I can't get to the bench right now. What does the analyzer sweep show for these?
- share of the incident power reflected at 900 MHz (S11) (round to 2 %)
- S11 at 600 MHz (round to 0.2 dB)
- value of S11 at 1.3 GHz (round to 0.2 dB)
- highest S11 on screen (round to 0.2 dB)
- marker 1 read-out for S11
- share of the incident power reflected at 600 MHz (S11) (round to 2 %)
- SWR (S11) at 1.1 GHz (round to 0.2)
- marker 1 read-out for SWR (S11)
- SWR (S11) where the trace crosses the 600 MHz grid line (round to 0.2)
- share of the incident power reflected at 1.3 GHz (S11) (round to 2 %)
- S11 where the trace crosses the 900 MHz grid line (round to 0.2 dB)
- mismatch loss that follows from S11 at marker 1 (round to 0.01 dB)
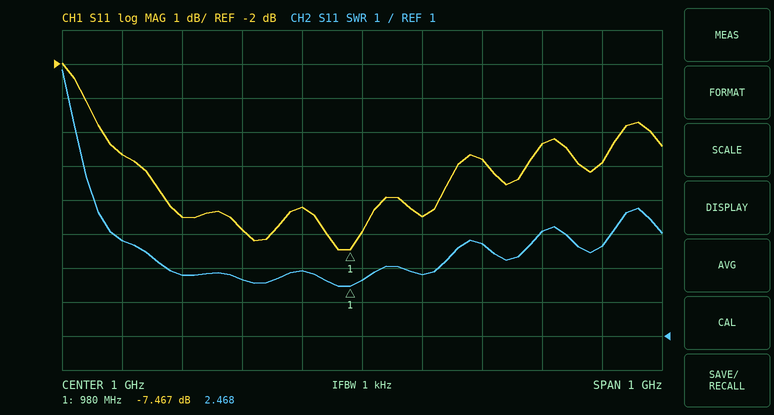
24 %
-4.6 dB
-4.4 dB
-2.0 dB
-7.467 dB
34 %
2.8
2.468
3.8
36 %
-6.2 dB
0.86 dB
